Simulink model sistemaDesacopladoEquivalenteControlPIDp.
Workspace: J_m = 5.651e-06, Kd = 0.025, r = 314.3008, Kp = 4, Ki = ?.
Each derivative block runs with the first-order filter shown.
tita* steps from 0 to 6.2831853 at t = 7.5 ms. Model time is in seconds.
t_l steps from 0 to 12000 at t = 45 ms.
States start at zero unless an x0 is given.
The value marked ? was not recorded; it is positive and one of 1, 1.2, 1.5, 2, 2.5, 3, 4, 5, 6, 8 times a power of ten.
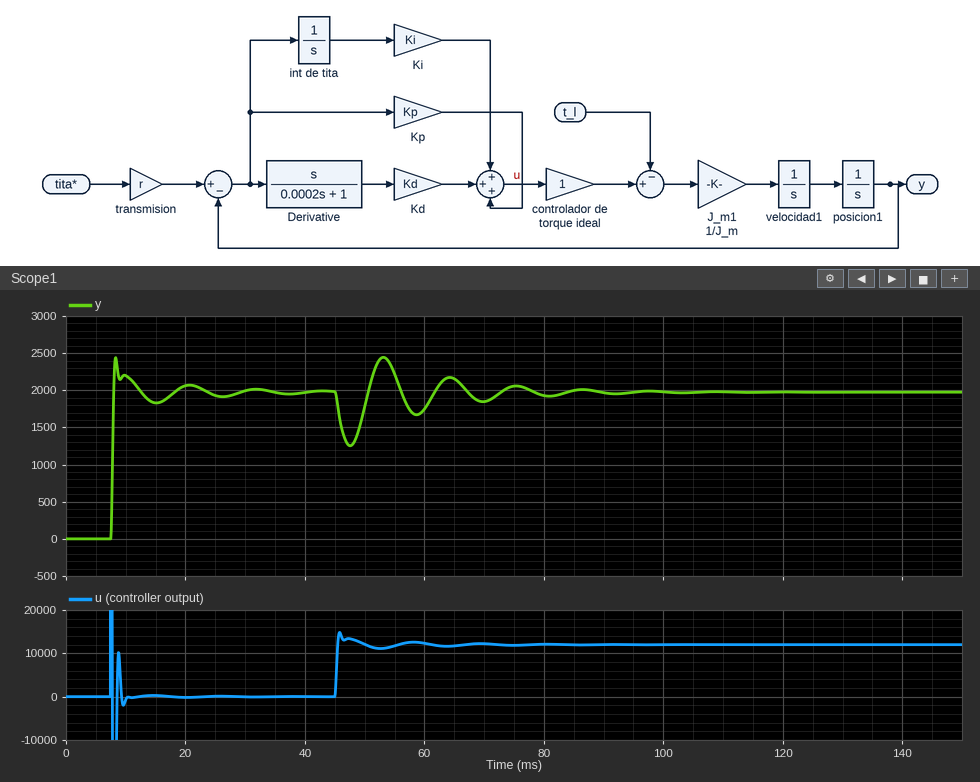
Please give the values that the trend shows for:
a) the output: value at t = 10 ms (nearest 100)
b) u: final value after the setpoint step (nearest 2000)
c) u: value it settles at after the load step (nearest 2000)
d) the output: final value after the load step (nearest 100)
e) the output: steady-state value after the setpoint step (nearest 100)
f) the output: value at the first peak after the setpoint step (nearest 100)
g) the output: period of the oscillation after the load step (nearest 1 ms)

2200
0
12000
2000
2000
2400
11 ms
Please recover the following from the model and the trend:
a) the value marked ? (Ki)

8000
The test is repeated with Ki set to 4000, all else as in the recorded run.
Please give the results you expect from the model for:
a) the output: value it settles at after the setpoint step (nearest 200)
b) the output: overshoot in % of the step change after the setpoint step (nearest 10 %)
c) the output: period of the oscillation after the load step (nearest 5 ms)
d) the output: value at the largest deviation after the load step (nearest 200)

2000
20 %
15 ms
1000
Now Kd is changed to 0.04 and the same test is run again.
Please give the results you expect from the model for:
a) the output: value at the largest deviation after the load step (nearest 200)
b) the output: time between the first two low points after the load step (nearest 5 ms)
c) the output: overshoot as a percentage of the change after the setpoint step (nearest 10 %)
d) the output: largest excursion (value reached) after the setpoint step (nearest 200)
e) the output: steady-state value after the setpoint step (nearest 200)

1400
15 ms
30 %
2600
2000
